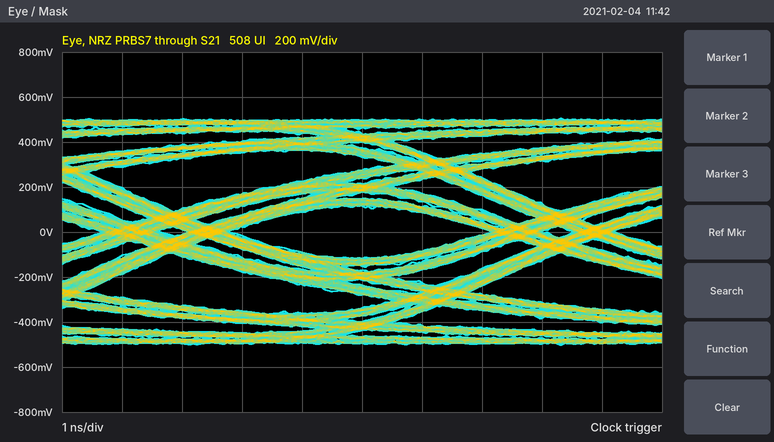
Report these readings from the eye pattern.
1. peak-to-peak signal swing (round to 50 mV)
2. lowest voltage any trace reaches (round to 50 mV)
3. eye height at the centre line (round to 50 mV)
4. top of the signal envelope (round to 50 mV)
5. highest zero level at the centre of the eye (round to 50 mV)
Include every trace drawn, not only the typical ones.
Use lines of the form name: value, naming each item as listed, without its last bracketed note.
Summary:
peak-to-peak signal swing: 1.00 V
lowest voltage any trace reaches: -500 mV
eye height at the centre line: 250 mV
top of the signal envelope: 500 mV
highest zero level at the centre of the eye: -100 mV
